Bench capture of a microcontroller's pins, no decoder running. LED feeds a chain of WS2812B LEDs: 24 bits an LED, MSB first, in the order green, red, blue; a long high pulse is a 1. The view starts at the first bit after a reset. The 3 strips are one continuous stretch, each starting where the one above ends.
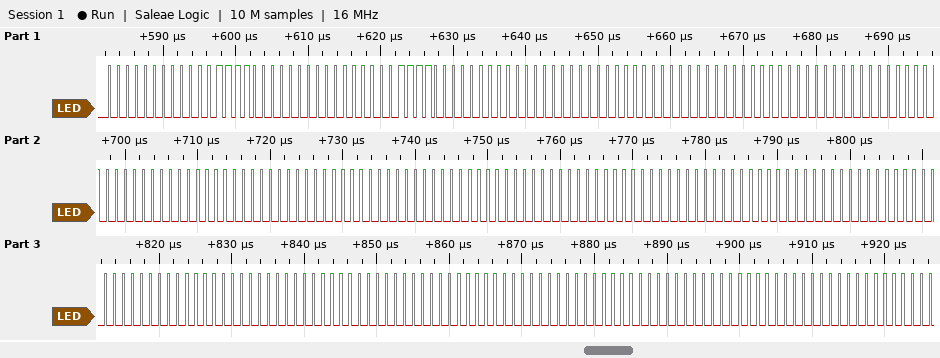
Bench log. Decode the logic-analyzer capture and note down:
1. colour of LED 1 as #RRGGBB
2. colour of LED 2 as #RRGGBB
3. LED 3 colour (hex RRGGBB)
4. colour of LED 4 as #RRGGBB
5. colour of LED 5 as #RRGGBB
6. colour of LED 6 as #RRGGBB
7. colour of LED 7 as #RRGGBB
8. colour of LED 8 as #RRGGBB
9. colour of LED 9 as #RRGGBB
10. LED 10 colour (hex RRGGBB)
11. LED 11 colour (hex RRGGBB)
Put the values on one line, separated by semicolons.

#0F0000; #F00000; #000000; #000000; #000000; #000000; #000000; #000000; #000000; #000000; #000000
